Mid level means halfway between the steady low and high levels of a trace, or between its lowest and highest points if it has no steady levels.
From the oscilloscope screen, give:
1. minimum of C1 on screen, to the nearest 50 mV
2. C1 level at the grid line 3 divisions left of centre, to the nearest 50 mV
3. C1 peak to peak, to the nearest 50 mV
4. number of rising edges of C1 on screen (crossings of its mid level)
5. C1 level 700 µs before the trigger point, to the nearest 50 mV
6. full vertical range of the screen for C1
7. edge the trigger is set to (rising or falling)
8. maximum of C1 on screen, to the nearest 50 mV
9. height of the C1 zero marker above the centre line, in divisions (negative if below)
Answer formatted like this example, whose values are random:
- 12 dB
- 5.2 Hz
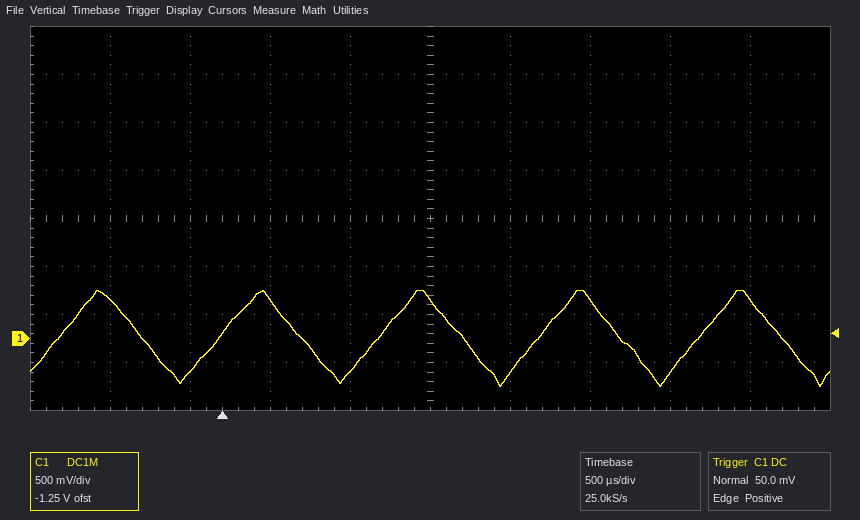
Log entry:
- -500 mV
- -350 mV
- 1.00 V
- 5
- 400 mV
- 4 V
- rising
- 500 mV
- -2.5 div
